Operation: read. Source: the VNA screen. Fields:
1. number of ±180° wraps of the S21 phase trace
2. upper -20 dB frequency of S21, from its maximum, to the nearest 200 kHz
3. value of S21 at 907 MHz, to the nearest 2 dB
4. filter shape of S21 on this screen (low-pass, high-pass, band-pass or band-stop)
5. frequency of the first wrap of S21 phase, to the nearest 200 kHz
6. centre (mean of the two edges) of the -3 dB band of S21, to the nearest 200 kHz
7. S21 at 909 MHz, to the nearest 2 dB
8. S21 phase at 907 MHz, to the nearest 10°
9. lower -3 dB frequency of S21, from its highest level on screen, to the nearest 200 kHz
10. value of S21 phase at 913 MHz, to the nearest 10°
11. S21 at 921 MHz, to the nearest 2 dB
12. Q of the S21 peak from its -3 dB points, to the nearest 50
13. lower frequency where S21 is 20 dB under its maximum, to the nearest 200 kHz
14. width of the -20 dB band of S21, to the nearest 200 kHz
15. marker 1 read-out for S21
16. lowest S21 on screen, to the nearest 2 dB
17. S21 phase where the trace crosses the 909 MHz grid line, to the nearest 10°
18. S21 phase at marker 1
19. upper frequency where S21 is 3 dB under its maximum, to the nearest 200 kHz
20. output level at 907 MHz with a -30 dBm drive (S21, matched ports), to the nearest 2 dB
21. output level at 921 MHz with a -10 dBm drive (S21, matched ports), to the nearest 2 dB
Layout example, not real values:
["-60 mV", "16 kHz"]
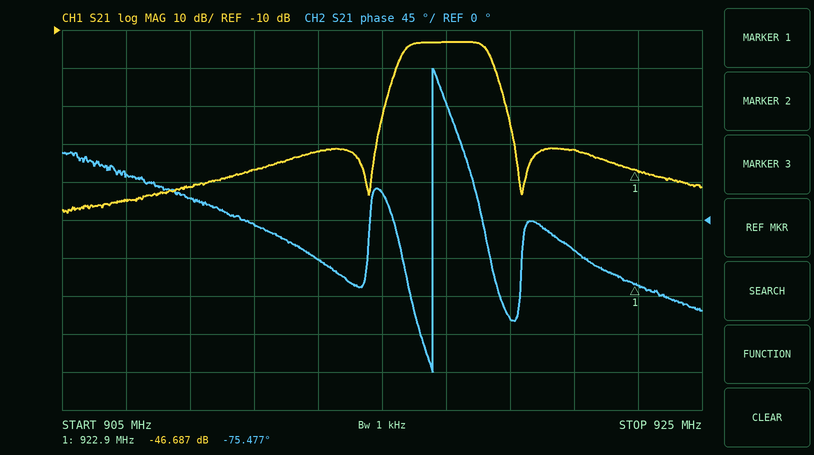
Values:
["1", "919.0 MHz", "-54 dB", "band-pass", "916.6 MHz", "917.0 MHz", "-52 dB", "50°", "915.6 MHz", "-50°", "-42 dB", "350", "915.0 MHz", "4.0 MHz", "-46.687 dB", "-58 dB", "30°", "-75.477°", "918.4 MHz", "-84 dBm", "-52 dBm"]
